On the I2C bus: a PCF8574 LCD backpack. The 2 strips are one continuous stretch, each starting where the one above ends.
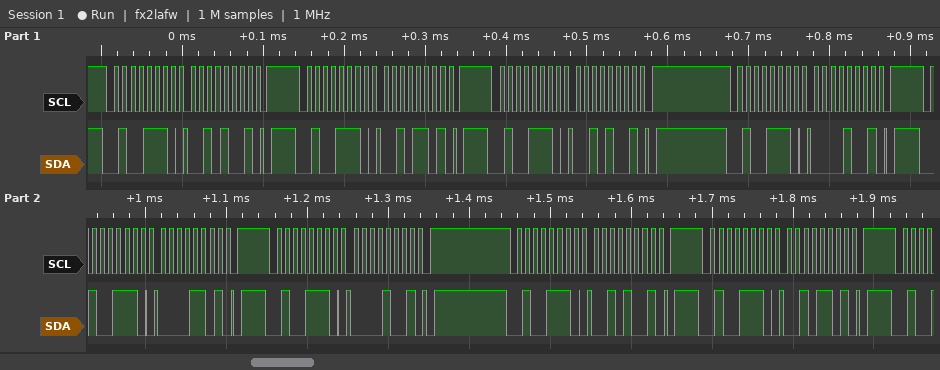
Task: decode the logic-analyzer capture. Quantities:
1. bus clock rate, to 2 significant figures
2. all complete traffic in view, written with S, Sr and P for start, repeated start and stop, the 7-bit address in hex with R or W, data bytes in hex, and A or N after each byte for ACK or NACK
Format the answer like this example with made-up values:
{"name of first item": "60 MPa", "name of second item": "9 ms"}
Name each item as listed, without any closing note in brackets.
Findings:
{"bus clock rate, to 2 significant figures": "100 kHz", "all complete traffic in view, written with S, Sr and P for start, repeated start and stop, the 7-bit address in hex with R or W, data bytes in hex, and A or N after each byte for ACK or NACK": "S 27W A 29 A P S 27W A 2D A P S 27W A 29 A P S 27W A 09 A P S 27W A 0D A P S 27W A 09 A P S 27W A 29 A P S 27W A 2D A P"}
